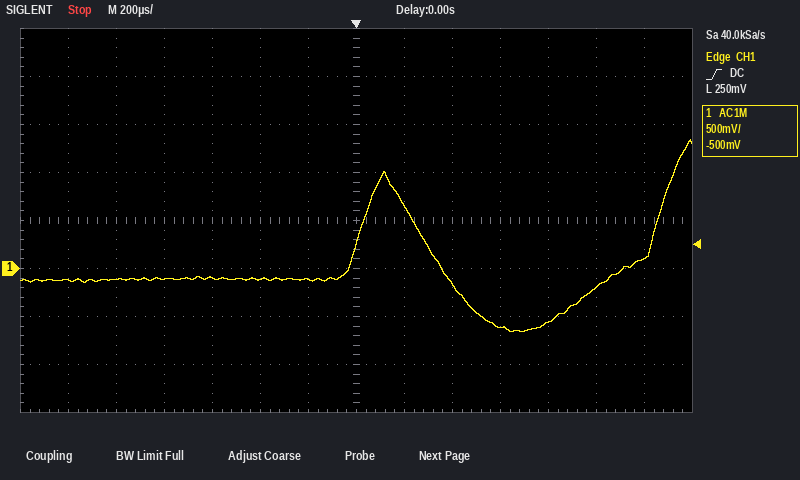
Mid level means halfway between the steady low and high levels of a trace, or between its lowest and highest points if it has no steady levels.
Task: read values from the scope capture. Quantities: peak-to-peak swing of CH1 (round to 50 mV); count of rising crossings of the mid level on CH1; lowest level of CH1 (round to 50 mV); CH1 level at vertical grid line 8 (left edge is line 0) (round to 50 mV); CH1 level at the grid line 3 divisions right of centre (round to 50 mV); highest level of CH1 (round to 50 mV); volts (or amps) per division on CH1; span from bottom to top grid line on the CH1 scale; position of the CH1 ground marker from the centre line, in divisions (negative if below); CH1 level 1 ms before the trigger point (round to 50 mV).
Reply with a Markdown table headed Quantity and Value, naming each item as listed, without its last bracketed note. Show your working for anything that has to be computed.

| Quantity | Value |
|---|---|
| peak-to-peak swing of CH1 | 1.35 V − (-650 mV) = 2.00 V |
| count of rising crossings of the mid level on CH1 | 2 |
| lowest level of CH1 | -650 mV |
| CH1 level at vertical grid line 8 (left edge is line 0) | 650 mV |
| CH1 level at the grid line 3 divisions right of centre | -600 mV |
| highest level of CH1 | 1.35 V |
| volts (or amps) per division on CH1 | 500 mV |
| span from bottom to top grid line on the CH1 scale | 4 V |
| position of the CH1 ground marker from the centre line, in divisions | -1.0 div |
| CH1 level 1 ms before the trigger point | -100 mV |
